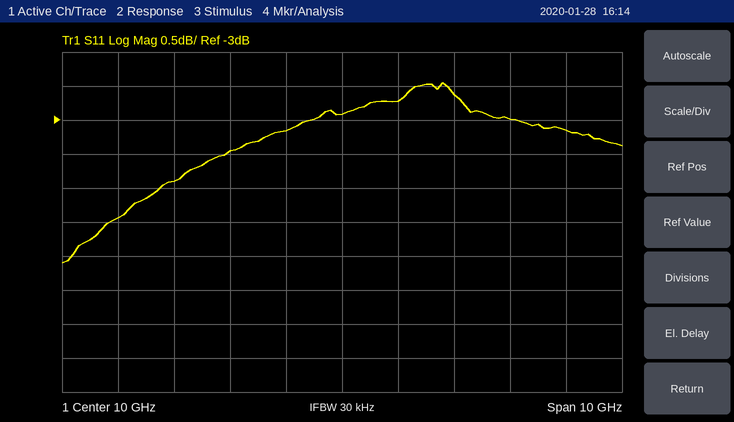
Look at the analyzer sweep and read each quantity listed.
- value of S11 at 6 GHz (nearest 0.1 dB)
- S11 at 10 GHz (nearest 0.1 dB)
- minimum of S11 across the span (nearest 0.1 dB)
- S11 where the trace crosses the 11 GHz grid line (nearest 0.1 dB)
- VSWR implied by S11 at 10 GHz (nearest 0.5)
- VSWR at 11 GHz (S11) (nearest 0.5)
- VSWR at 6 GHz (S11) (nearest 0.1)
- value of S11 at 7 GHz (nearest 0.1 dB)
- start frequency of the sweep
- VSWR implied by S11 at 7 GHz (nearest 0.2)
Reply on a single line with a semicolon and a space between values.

-4.4 dB; -2.9 dB; -5.1 dB; -2.7 dB; 6.0; 6.5; 4.0; -3.9 dB; 5 GHz; 4.6
